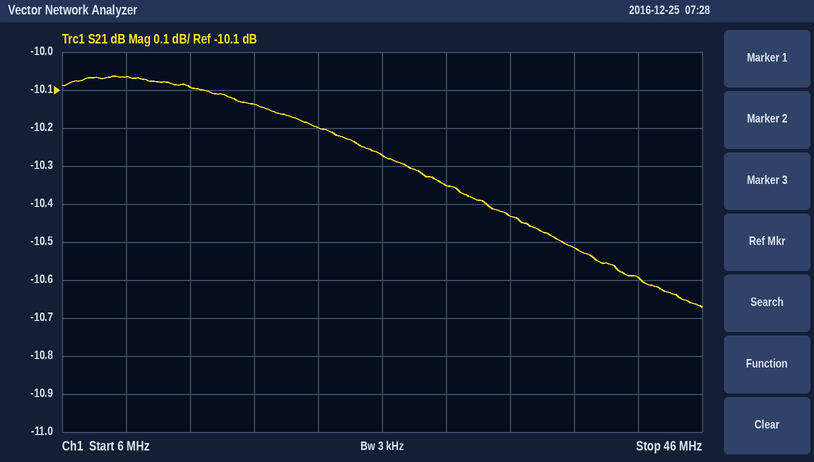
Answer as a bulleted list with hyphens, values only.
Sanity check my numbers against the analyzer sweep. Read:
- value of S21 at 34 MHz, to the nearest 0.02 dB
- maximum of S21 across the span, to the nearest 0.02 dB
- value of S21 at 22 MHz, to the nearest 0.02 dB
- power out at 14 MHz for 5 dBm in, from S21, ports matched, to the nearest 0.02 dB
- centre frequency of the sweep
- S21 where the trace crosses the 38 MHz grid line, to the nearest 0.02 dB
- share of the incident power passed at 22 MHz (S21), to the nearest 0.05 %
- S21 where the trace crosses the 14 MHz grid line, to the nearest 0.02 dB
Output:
- -10.44 dB
- -10.06 dB
- -10.20 dB
- -5.10 dBm
- 26 MHz
- -10.52 dB
- 9.55 %
- -10.10 dB
